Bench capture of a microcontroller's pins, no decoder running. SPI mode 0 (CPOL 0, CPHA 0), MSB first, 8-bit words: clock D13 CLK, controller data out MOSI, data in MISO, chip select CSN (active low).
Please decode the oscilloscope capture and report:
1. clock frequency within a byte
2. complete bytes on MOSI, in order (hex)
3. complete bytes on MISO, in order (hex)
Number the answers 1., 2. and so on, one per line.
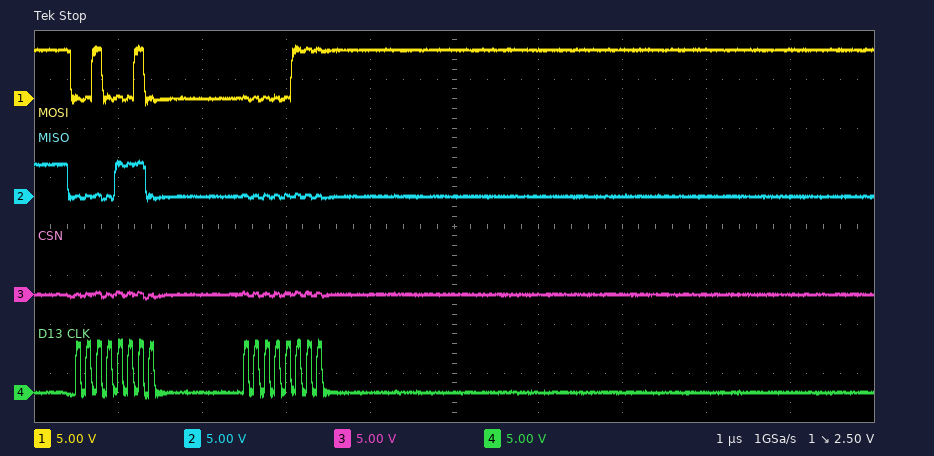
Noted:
1. 8 MHz
2. 22 07
3. 0E 00
